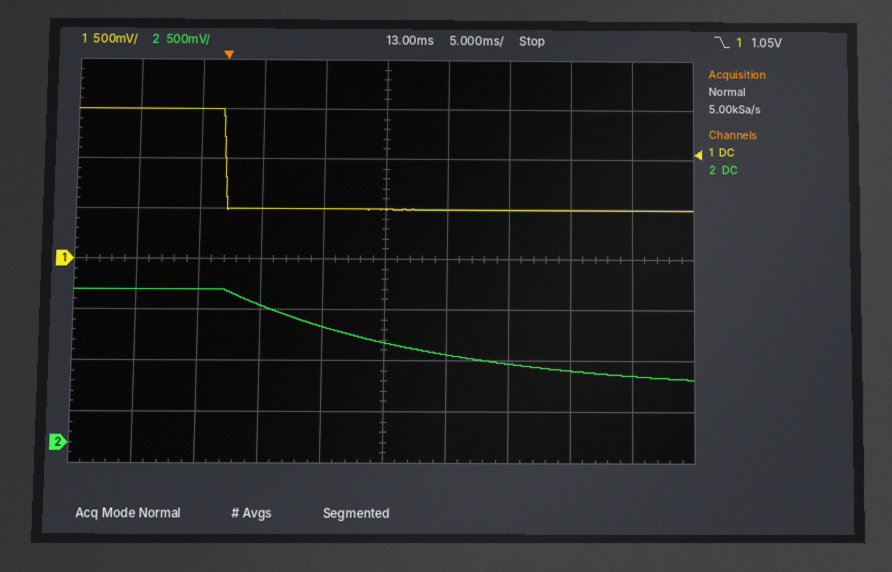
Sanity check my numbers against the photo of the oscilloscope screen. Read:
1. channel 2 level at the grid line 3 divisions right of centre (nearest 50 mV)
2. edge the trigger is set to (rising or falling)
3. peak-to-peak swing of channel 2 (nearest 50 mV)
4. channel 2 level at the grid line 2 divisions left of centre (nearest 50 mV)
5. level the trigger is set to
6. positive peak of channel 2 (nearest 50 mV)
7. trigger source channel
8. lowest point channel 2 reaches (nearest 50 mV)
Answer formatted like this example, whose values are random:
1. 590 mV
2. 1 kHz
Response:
1. 700 mV
2. falling
3. 900 mV
4. 1.35 V
5. 1.05 V
6. 1.50 V
7. channel 1
8. 600 mV
